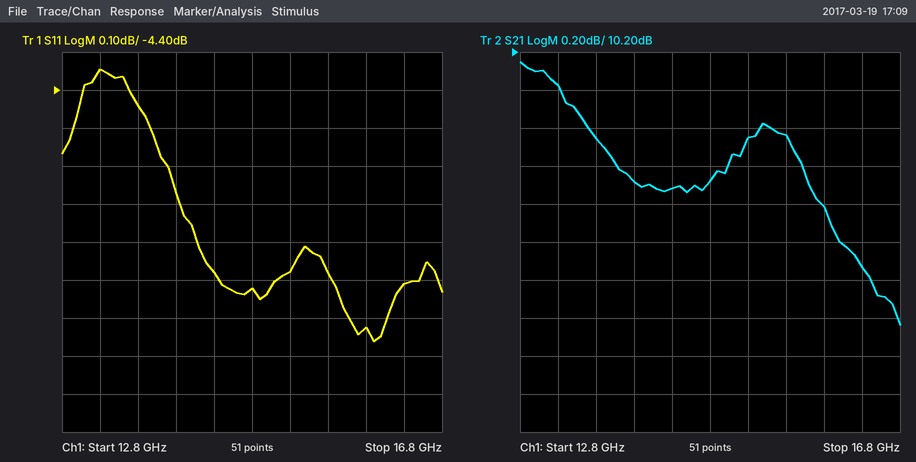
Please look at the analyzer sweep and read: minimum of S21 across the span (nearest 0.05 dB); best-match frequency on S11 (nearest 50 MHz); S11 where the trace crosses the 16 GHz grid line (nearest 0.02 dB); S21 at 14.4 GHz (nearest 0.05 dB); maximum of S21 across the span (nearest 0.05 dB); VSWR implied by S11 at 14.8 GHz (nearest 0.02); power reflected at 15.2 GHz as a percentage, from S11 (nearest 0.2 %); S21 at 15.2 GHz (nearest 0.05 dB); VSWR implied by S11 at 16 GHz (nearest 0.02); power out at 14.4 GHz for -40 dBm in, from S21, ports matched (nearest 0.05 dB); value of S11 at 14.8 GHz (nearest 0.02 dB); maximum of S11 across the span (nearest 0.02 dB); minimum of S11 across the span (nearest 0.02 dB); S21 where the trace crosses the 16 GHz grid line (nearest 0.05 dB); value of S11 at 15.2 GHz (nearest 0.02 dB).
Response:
8.75 dB
16.10 GHz
-5.02 dB
9.50 dB
10.15 dB
3.62
32.6 %
9.75 dB
3.56
-30.50 dBm
-4.92 dB
-4.34 dB
-5.06 dB
9.40 dB
-4.88 dB
